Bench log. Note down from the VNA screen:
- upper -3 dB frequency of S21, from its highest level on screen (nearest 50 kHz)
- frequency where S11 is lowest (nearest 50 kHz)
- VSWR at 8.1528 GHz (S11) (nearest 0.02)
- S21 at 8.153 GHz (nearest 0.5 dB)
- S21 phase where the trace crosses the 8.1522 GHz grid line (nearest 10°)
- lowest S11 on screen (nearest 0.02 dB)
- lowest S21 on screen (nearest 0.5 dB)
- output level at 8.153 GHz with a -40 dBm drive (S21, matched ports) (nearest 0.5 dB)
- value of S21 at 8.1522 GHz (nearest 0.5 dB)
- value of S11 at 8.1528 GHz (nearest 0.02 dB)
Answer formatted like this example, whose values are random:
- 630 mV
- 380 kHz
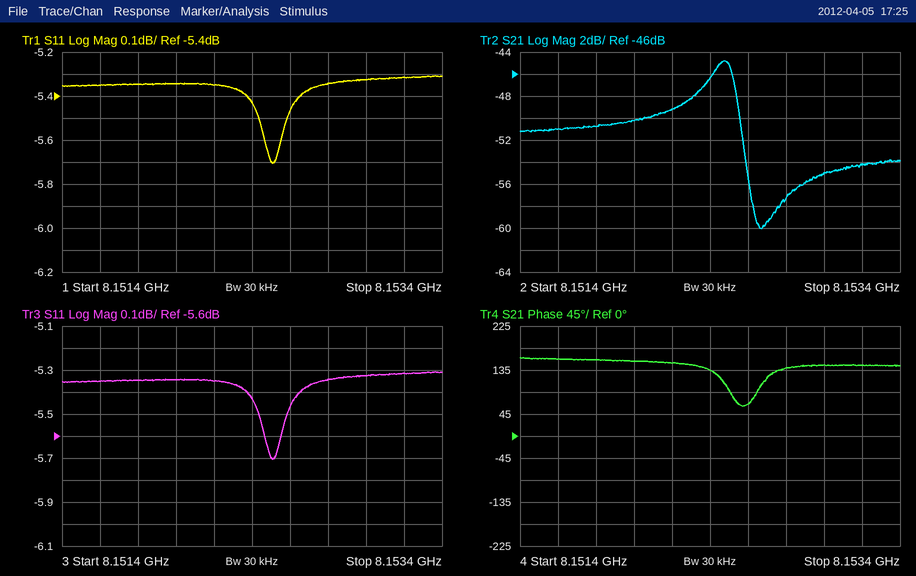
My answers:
- 8.15255 GHz
- 8.15250 GHz
- 3.36
- -55.0 dB
- 150°
- -5.70 dB
- -60.0 dB
- -95.0 dBm
- -49.0 dB
- -5.34 dB
